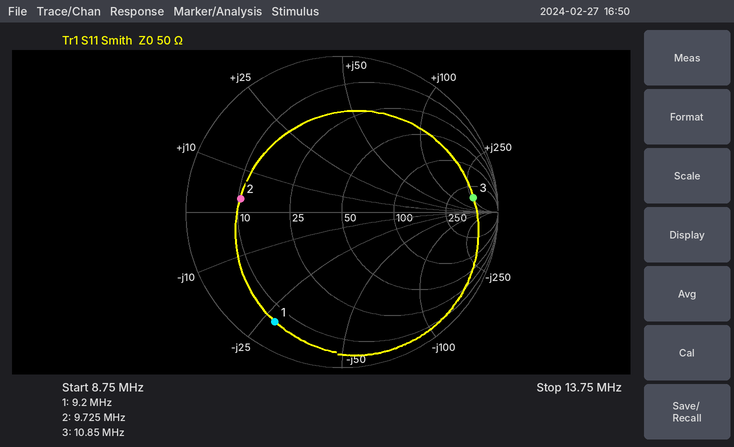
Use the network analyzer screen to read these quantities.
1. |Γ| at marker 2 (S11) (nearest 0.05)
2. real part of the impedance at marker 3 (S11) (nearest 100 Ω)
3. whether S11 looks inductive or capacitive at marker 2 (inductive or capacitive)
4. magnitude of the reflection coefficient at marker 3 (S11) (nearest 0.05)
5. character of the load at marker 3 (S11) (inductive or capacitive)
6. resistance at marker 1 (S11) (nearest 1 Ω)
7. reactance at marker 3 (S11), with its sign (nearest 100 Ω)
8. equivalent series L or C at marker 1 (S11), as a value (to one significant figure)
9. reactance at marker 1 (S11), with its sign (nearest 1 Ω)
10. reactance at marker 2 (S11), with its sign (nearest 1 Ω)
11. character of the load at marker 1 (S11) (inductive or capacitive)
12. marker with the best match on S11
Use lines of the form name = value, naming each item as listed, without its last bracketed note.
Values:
|Γ| at marker 2 (S11) = 0.65
real part of the impedance at marker 3 (S11) = 400 Ω
whether S11 looks inductive or capacitive at marker 2 = inductive
magnitude of the reflection coefficient at marker 3 (S11) = 0.85
character of the load at marker 3 (S11) = inductive
resistance at marker 1 (S11) = 6 Ω
reactance at marker 3 (S11), with its sign = +300 Ω
equivalent series L or C at marker 1 (S11), as a value = 600 pF
reactance at marker 1 (S11), with its sign = -28 Ω
reactance at marker 2 (S11), with its sign = +3 Ω
character of the load at marker 1 (S11) = capacitive
marker with the best match on S11 = marker 2
